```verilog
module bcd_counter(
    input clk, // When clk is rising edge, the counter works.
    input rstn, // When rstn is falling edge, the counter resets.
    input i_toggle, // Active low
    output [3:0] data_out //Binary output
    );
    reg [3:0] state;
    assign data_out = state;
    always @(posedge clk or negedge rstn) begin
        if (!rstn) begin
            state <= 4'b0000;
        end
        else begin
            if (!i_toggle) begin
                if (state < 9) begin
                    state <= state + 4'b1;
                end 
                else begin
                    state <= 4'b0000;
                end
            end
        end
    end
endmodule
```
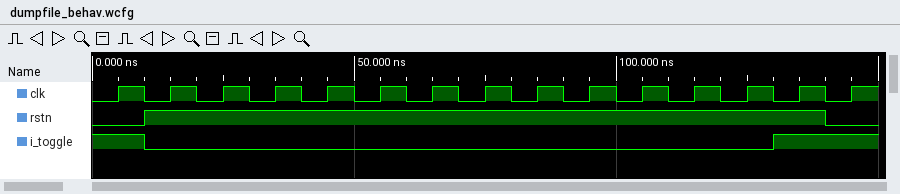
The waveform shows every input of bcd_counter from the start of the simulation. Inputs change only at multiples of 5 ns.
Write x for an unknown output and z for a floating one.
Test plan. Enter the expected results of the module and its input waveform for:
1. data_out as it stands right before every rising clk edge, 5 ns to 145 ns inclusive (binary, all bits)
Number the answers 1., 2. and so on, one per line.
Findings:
1. 0000, 0000, 0001, 0010, 0011, 0100, 0101, 0110, 0111, 1000, 1001, 0000, 0001, 0010, 0000
